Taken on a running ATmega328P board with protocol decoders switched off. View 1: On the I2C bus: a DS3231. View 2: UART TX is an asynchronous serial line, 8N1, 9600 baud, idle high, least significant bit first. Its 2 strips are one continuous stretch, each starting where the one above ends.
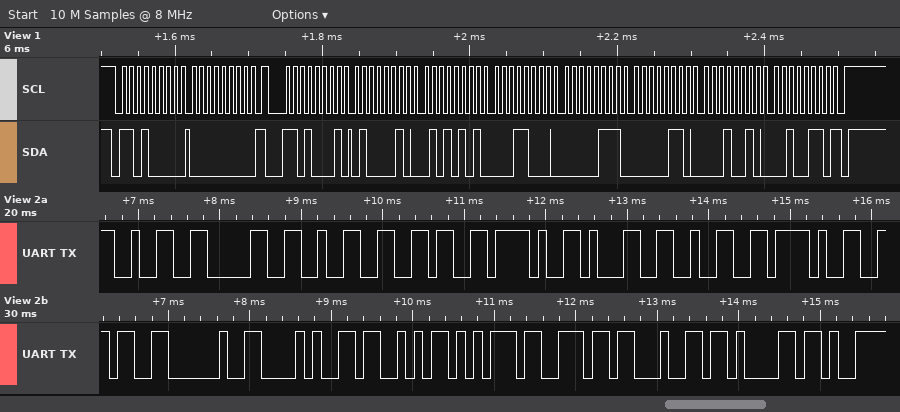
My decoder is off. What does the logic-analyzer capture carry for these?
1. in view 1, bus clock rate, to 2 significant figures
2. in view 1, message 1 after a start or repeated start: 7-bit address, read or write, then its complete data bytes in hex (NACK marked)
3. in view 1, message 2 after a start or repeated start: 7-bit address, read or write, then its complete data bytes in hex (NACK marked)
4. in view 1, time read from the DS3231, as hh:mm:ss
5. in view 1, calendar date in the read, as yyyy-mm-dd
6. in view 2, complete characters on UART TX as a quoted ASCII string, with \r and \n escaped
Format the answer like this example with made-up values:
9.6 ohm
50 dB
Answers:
100 kHz
0x68 write: 00
0x68 read: 42 55 18 07 06 12 26 NACK
18:55:42
2026-12-06
"2026/12/6 (Sunda"
